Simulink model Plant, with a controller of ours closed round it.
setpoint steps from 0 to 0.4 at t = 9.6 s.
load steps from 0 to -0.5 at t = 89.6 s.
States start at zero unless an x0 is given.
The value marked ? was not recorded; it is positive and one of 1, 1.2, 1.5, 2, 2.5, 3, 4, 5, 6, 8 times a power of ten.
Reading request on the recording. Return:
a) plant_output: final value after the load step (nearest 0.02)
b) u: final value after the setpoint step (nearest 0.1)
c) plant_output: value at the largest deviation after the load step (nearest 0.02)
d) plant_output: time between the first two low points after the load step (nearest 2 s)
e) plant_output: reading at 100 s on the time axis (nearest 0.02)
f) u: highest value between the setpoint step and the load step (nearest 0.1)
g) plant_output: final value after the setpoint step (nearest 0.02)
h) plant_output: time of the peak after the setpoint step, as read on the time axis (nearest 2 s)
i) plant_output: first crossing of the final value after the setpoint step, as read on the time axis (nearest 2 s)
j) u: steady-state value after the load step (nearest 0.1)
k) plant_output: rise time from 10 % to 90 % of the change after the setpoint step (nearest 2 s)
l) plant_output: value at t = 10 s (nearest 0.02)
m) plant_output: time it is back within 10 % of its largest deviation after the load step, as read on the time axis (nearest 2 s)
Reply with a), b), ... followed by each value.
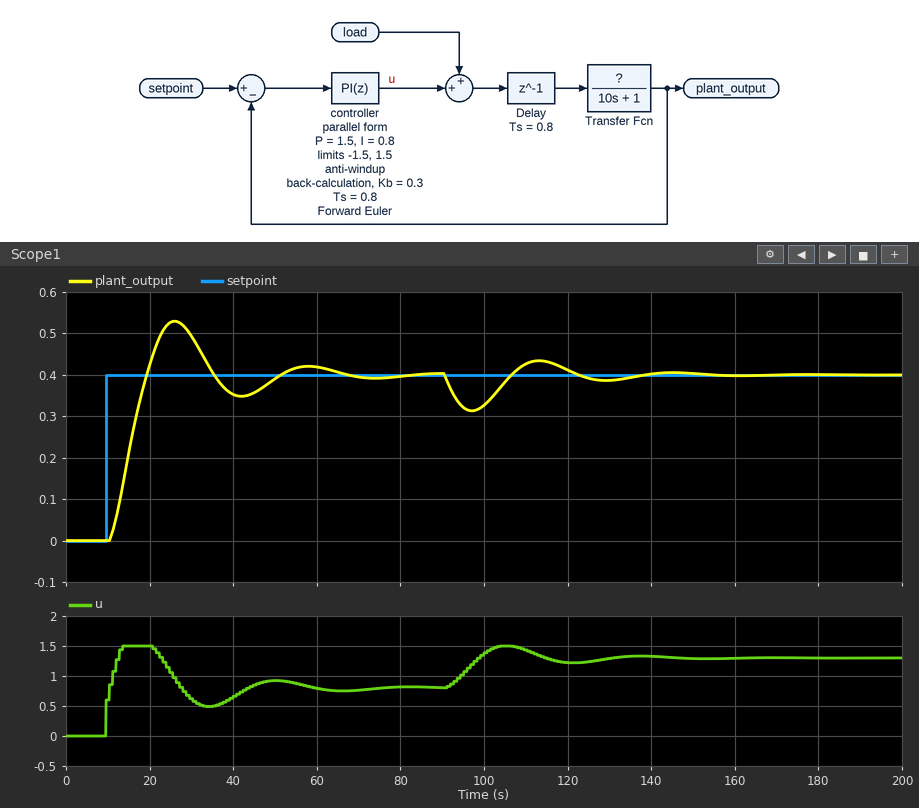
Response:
a) 0.40
b) 0.8
c) 0.32
d) 32 s
e) 0.32
f) 1.5
g) 0.40
h) 26 s
i) 20 s
j) 1.3
k) 6 s
l) 0.00
m) 134 s
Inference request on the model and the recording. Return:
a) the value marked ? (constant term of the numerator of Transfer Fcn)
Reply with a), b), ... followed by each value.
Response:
a) 0.5
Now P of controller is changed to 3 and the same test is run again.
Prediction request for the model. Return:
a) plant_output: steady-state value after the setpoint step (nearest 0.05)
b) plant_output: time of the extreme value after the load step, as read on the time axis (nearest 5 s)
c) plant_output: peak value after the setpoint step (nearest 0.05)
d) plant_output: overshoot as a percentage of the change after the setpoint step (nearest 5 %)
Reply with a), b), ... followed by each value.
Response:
a) 0.40
b) 95 s
c) 0.50
d) 20 %
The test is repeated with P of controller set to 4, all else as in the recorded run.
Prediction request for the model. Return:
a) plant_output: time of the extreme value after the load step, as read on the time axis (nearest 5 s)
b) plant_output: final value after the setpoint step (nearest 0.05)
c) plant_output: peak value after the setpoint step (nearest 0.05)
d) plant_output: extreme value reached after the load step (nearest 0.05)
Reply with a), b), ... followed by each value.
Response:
a) 95 s
b) 0.40
c) 0.45
d) 0.35
